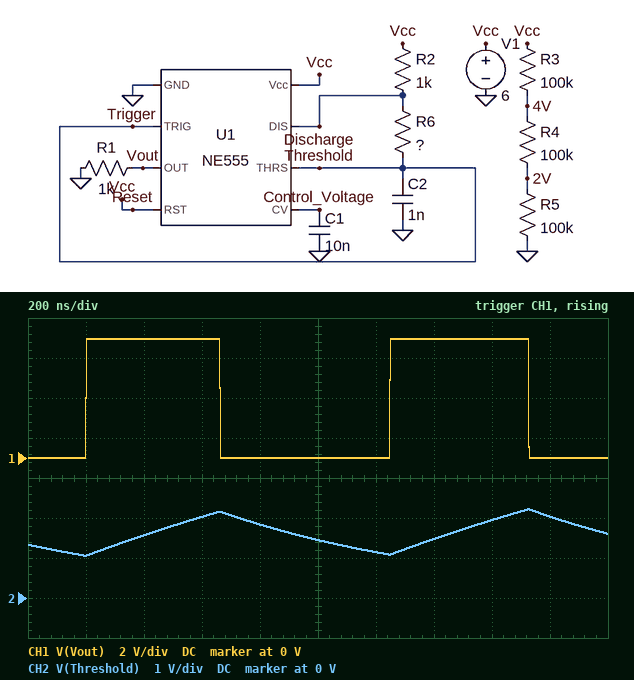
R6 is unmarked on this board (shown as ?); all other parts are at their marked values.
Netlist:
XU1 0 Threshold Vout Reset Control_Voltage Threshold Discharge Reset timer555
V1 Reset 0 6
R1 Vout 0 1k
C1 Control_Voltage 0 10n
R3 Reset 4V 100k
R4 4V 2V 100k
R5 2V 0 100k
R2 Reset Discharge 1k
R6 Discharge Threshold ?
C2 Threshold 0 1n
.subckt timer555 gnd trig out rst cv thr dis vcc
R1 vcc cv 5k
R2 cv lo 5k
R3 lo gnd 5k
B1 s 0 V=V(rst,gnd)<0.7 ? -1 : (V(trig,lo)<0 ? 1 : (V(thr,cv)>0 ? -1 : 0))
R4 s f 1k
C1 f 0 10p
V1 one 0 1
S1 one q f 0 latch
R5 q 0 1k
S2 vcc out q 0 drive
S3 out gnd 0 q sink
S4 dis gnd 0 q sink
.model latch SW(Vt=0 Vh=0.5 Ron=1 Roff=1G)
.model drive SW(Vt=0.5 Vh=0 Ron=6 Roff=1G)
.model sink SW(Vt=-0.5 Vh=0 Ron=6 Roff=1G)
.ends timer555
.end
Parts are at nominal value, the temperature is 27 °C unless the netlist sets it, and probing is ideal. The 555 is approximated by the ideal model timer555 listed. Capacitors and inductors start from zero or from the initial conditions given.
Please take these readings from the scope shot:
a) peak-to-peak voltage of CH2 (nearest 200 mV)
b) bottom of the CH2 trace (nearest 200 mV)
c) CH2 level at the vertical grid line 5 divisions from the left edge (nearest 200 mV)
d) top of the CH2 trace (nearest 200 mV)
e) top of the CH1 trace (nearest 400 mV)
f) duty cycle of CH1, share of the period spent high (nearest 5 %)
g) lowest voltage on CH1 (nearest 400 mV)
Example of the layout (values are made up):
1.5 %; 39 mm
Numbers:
1.2 V; 1.0 V; 1.4 V; 2.2 V; 6.0 V; 45 %; 0 V
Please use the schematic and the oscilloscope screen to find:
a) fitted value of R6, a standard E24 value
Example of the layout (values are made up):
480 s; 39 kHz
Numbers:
820 Ω
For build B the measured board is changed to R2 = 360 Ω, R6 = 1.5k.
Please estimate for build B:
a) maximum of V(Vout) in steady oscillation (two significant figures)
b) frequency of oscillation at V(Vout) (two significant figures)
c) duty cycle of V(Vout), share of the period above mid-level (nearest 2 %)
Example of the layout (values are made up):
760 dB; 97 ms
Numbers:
6.0 V; 630 kHz; 32 %
